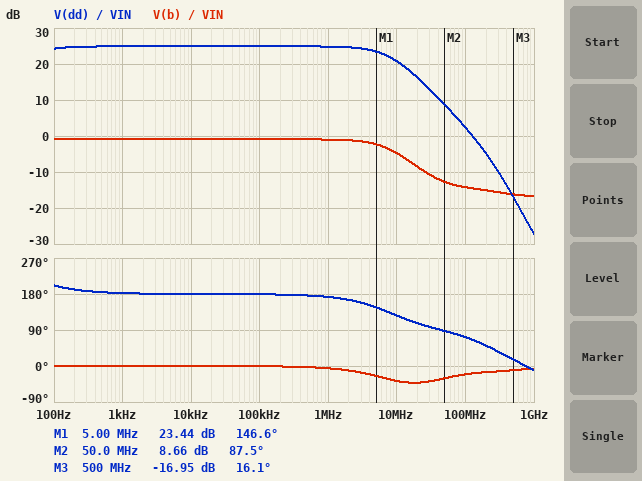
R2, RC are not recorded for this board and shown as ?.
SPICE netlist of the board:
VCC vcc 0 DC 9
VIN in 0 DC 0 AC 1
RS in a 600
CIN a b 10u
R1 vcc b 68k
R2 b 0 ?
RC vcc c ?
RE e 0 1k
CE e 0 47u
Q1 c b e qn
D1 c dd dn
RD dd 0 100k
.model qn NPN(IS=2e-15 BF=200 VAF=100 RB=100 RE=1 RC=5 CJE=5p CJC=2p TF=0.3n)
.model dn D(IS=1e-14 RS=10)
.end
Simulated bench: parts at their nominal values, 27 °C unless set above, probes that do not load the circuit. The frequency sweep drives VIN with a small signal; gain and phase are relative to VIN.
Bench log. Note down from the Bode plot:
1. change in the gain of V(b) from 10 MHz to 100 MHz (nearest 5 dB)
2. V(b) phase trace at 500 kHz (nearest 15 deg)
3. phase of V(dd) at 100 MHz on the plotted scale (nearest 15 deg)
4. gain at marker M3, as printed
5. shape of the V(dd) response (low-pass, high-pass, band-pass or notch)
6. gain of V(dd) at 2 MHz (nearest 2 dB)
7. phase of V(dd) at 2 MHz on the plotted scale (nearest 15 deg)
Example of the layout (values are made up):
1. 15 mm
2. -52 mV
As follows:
1. -10 dB
2. 0 deg
3. 75 deg
4. -16.95 dB
5. low-pass
6. 24 dB
7. 165 deg
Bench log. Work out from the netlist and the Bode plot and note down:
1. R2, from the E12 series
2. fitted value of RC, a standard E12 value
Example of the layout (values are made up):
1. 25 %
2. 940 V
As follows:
1. 8.2 kΩ
2. 1.8 kΩ
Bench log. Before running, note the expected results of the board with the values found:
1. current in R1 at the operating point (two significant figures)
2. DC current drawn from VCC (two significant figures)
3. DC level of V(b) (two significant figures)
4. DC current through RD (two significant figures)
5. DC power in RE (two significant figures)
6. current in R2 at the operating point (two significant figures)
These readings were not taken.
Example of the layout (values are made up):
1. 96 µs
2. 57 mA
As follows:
1. 120 µA
2. 490 µA
3. 960 mV
4. 77 µA
5. 87 µW
6. 120 µA
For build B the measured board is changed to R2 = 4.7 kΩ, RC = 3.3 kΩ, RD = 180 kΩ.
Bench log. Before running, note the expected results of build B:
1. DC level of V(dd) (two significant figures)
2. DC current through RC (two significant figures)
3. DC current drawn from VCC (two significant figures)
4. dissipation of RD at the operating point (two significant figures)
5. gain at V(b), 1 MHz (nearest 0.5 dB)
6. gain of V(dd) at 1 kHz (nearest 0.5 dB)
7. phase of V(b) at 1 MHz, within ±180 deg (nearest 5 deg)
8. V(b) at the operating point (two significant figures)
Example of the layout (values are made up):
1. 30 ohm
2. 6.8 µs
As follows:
1. 8.2 V
2. 55 µA
3. 180 µA
4. 380 µW
5. -1.0 dB
6. 0 dB
7. 0 deg
8. 580 mV
